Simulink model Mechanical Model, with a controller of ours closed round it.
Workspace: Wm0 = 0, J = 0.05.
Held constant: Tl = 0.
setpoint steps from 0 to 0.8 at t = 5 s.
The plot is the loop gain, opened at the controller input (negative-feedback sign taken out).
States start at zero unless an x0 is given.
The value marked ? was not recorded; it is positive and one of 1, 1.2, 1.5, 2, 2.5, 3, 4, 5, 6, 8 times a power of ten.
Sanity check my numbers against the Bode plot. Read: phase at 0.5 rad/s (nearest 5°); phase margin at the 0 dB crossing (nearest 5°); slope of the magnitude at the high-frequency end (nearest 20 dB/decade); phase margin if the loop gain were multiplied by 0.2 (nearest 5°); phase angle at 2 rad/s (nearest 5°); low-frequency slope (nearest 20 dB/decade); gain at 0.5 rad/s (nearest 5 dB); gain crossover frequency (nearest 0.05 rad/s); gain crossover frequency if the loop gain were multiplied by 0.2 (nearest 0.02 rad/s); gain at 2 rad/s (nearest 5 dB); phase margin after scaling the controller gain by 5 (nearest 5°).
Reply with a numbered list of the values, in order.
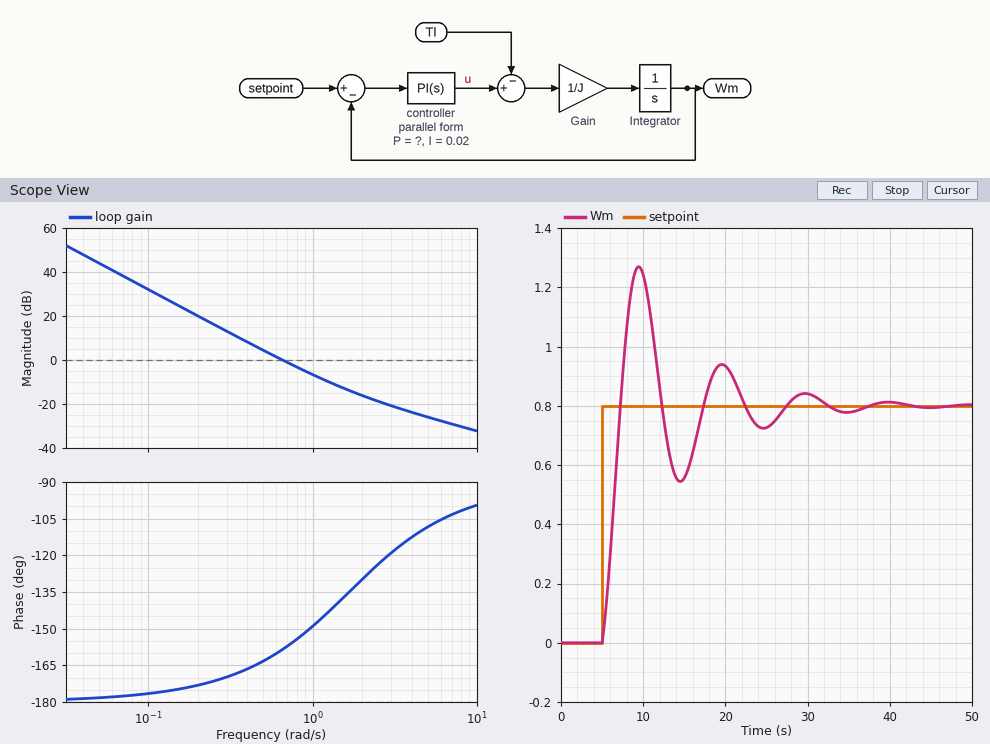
1. -165°
2. 20°
3. -20 dB/decade
4. 10°
5. -130°
6. -40 dB/decade
7. 5 dB
8. 0.65 rad/s
9. 0.28 rad/s
10. -15 dB
11. 45°
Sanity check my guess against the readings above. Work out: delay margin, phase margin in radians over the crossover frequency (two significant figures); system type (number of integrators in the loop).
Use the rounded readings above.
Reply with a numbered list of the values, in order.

1. 0.54 s
2. 2
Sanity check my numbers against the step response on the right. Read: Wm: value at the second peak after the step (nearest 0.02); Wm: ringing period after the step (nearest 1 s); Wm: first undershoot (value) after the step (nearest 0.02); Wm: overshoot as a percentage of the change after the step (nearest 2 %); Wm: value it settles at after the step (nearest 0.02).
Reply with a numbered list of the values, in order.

1. 0.94
2. 10 s
3. 0.54
4. 58 %
5. 0.80
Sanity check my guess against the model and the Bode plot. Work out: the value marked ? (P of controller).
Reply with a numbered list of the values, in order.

1. 0.012
